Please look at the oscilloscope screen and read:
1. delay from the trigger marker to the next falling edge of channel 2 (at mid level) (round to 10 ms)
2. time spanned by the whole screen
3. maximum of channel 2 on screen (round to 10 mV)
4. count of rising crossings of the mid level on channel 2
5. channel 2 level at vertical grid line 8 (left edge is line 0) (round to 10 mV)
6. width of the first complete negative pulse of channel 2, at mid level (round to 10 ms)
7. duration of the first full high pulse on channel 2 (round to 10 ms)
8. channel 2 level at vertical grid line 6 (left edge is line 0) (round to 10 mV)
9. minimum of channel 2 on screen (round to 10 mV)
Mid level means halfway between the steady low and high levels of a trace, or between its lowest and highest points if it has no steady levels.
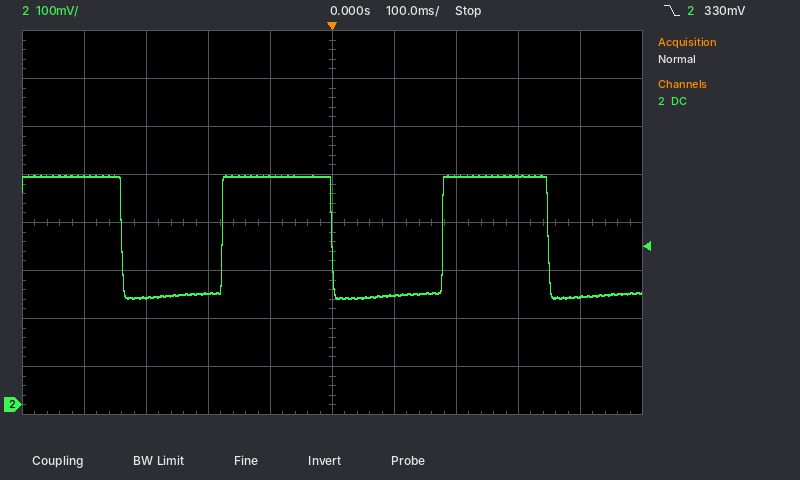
350 ms
1 s
480 mV
2
480 mV
160 ms
180 ms
230 mV
220 mV
